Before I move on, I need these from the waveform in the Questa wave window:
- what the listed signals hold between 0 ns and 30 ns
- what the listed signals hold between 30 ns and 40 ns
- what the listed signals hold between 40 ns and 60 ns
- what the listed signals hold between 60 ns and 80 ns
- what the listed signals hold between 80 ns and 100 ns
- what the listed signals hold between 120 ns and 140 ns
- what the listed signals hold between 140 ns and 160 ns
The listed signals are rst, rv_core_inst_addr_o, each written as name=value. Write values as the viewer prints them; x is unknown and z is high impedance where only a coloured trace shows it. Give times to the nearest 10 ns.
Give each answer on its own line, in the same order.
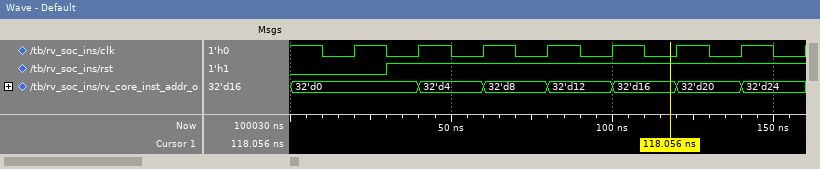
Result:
rst=0, rv_core_inst_addr_o=32'd0
rst=1, rv_core_inst_addr_o=32'd0
rst=1, rv_core_inst_addr_o=32'd4
rst=1, rv_core_inst_addr_o=32'd8
rst=1, rv_core_inst_addr_o=32'd12
rst=1, rv_core_inst_addr_o=32'd20
rst=1, rv_core_inst_addr_o=32'd24
